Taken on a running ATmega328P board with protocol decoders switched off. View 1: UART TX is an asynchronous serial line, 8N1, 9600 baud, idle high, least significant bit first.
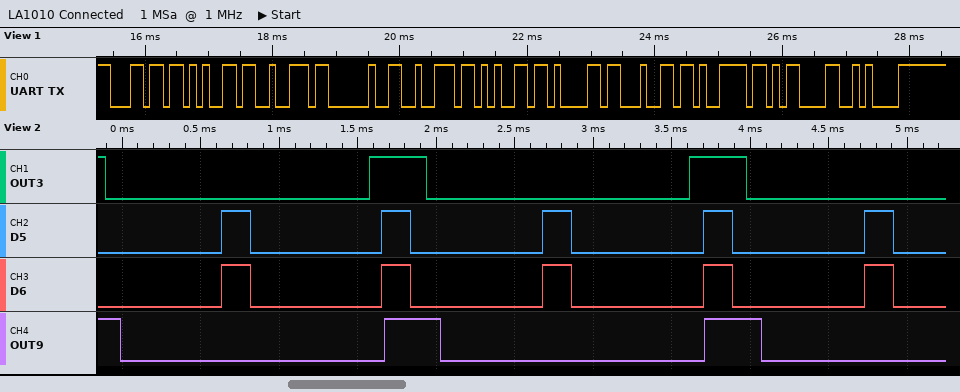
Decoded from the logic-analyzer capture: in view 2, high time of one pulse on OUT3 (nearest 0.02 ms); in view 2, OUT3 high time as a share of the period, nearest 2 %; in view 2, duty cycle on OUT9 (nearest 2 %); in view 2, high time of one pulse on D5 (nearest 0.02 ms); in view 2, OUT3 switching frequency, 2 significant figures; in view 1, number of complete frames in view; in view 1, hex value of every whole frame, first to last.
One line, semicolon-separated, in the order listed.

0.36 ms; 18 %; 18 %; 0.18 ms; 490 Hz; 11; 0x6C 0x65 0x72 0x20 0x72 0x65 0x61 0x64 0x79 0x0D 0x0A
